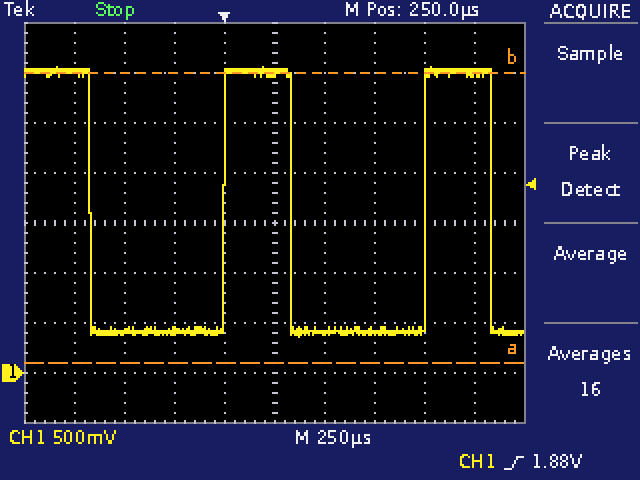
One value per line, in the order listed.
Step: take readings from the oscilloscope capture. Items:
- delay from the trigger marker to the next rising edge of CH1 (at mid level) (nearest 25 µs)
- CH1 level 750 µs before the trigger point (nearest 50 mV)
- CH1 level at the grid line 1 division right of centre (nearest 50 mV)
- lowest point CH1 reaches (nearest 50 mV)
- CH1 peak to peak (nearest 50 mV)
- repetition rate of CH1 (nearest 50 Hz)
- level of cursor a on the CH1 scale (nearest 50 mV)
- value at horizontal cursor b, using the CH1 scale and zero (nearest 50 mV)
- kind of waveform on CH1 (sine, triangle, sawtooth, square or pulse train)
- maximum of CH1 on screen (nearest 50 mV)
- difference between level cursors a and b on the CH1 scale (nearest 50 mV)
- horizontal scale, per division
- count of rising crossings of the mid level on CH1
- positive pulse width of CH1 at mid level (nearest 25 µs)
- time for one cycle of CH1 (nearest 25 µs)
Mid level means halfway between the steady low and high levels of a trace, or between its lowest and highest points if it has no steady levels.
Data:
1.000 ms
3.00 V
400 mV
350 mV
2.70 V
1.00 kHz
100 mV
3.00 V
pulse train
3.05 V
2.90 V
250 µs
2
325 µs
1.000 ms
